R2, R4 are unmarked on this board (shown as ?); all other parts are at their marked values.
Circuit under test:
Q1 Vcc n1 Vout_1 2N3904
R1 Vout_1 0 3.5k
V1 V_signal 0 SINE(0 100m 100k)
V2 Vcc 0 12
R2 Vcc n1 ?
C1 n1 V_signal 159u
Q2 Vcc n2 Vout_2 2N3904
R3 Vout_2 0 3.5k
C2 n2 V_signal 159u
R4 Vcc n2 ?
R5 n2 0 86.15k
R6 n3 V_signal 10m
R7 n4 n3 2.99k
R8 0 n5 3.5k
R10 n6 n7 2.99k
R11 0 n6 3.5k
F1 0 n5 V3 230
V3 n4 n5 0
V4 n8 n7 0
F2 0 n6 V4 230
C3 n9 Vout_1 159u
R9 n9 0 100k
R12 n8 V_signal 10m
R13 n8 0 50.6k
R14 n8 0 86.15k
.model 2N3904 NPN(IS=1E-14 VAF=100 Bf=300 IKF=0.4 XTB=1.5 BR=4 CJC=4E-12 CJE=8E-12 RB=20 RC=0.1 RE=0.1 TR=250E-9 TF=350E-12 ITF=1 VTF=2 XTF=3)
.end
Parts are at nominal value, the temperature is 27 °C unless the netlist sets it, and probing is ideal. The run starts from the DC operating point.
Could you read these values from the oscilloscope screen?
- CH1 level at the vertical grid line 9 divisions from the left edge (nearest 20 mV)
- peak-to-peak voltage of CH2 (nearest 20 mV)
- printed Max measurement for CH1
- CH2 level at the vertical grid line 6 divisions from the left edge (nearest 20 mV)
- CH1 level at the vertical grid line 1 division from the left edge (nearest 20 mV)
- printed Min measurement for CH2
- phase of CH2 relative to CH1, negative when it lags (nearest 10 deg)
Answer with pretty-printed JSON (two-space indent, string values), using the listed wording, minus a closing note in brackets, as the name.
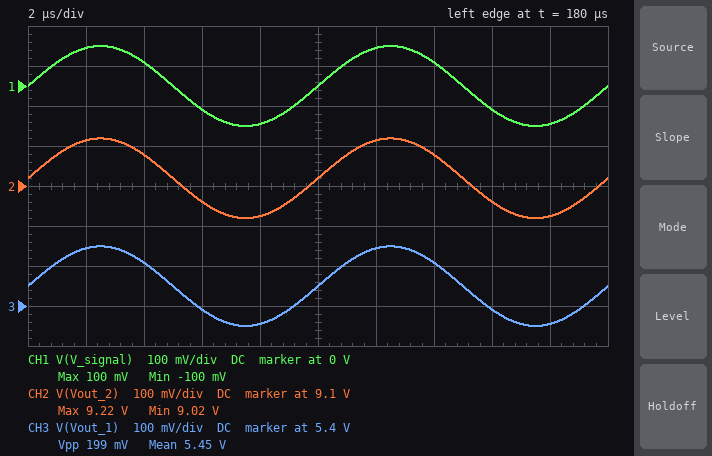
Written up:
{
  "CH1 level at the vertical grid line 9 divisions from the left edge": "-100 mV",
  "peak-to-peak voltage of CH2": "200 mV",
  "printed Max measurement for CH1": "100 mV",
  "CH2 level at the vertical grid line 6 divisions from the left edge": "9.22 V",
  "CH1 level at the vertical grid line 1 division from the left edge": "100 mV",
  "printed Min measurement for CH2": "9.02 V",
  "phase of CH2 relative to CH1, negative when it lags": "0 deg"
}
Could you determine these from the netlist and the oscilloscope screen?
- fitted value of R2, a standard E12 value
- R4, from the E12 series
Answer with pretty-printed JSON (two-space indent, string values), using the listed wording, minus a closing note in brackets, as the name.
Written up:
{
  "fitted value of R2, a standard E12 value": "1.2 MΩ",
  "R4, from the E12 series": "18 kΩ"
}
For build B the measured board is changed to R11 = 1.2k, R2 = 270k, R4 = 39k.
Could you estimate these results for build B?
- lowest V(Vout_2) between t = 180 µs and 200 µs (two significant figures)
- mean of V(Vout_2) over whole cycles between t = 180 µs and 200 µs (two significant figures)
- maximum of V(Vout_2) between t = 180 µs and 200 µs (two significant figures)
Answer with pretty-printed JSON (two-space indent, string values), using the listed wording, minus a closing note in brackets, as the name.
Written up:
{
  "lowest V(Vout_2) between t = 180 µs and 200 µs": "7.3 V",
  "mean of V(Vout_2) over whole cycles between t = 180 µs and 200 µs": "7.4 V",
  "maximum of V(Vout_2) between t = 180 µs and 200 µs": "7.5 V"
}
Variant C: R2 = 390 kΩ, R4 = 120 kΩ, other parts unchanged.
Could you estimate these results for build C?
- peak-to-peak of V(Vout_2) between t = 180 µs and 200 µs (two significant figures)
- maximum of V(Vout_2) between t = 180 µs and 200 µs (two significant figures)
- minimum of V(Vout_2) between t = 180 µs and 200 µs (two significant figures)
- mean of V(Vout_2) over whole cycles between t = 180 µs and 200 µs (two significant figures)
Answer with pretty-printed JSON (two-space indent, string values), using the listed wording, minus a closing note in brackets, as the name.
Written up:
{
  "peak-to-peak of V(Vout_2) between t = 180 µs and 200 µs": "200 mV",
  "maximum of V(Vout_2) between t = 180 µs and 200 µs": "4.3 V",
  "minimum of V(Vout_2) between t = 180 µs and 200 µs": "4.1 V",
  "mean of V(Vout_2) over whole cycles between t = 180 µs and 200 µs": "4.2 V"
}
